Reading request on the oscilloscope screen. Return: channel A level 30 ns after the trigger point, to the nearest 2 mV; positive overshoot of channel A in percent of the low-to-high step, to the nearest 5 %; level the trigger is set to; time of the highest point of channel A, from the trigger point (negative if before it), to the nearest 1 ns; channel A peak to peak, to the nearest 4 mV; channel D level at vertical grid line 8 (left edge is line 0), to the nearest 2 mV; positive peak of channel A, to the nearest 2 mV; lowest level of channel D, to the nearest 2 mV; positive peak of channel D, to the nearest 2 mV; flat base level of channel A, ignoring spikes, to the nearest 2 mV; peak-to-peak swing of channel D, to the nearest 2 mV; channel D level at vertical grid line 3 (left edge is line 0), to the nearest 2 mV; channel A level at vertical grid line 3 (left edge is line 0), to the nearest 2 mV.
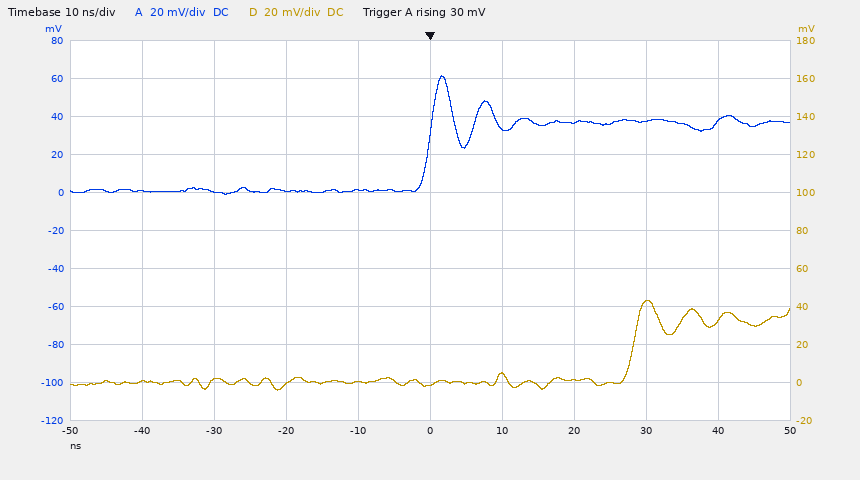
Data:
38 mV
65 %
30 mV
+2 ns
64 mV
42 mV
62 mV
-4 mV
44 mV
0 mV
48 mV
0 mV
0 mV
